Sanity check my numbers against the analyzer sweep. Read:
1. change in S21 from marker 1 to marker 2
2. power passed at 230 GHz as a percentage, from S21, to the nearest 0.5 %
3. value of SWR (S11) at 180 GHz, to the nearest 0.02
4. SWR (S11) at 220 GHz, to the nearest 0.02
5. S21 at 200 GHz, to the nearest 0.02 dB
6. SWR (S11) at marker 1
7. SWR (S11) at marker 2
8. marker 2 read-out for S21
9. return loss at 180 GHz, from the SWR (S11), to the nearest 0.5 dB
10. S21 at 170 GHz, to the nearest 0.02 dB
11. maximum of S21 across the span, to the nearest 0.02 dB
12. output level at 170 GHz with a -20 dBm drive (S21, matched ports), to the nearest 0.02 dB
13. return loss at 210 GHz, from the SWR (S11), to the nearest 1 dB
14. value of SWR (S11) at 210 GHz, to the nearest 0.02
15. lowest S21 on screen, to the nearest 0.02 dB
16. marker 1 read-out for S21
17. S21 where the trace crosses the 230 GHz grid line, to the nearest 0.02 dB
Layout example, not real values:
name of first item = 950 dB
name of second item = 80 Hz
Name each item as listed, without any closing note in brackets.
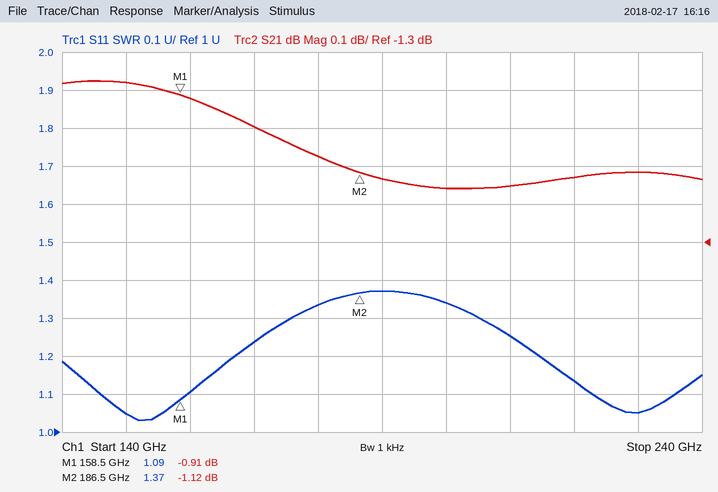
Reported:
change in S21 from marker 1 to marker 2 = -0.21 dB
power passed at 230 GHz as a percentage, from S21, to the nearest 0.5 % = 77.5 %
value of SWR (S11) at 180 GHz, to the nearest 0.02 = 1.34
SWR (S11) at 220 GHz, to the nearest 0.02 = 1.14
S21 at 200 GHz, to the nearest 0.02 dB = -1.16 dB
SWR (S11) at marker 1 = 1.09
SWR (S11) at marker 2 = 1.37
marker 2 read-out for S21 = -1.12 dB
return loss at 180 GHz, from the SWR (S11), to the nearest 0.5 dB = 17.0 dB
S21 at 170 GHz, to the nearest 0.02 dB = -1.00 dB
maximum of S21 across the span, to the nearest 0.02 dB = -0.88 dB
output level at 170 GHz with a -20 dBm drive (S21, matched ports), to the nearest 0.02 dB = -21.00 dBm
return loss at 210 GHz, from the SWR (S11), to the nearest 1 dB = 19 dB
value of SWR (S11) at 210 GHz, to the nearest 0.02 = 1.26
lowest S21 on screen, to the nearest 0.02 dB = -1.16 dB
marker 1 read-out for S21 = -0.91 dB
S21 where the trace crosses the 230 GHz grid line, to the nearest 0.02 dB = -1.12 dB
